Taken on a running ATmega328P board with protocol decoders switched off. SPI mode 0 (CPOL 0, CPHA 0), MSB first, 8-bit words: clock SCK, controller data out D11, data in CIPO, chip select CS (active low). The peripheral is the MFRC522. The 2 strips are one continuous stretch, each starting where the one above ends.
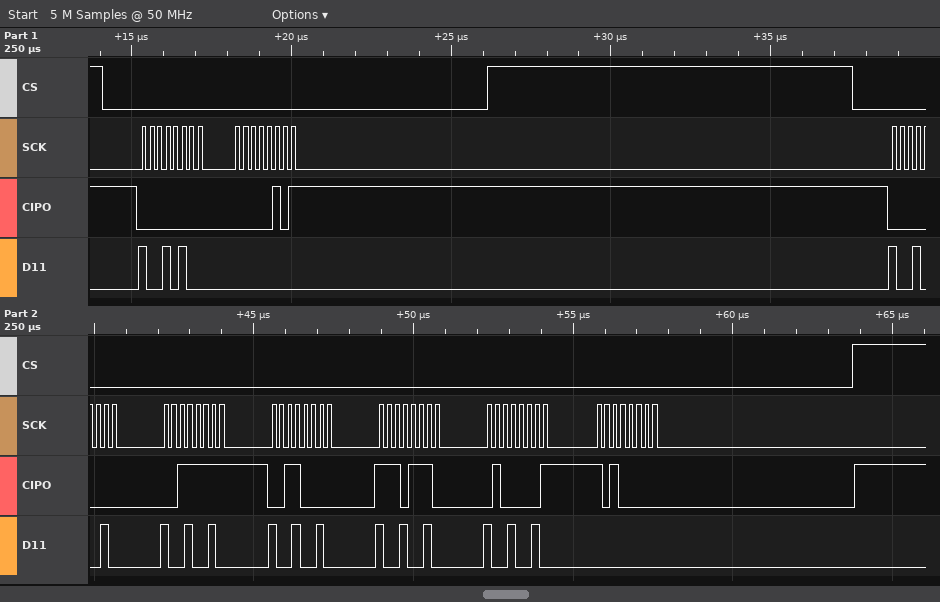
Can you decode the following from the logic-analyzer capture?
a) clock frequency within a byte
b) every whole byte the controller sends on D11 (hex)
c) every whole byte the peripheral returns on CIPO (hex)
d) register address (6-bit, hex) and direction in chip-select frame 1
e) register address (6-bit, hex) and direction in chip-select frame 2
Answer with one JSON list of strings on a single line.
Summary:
["4 MHz", "94 00 92 92 92 92 92 00", "00 05 00 3F 30 EE 41 A0", "0x0A read", "0x09 read"]
